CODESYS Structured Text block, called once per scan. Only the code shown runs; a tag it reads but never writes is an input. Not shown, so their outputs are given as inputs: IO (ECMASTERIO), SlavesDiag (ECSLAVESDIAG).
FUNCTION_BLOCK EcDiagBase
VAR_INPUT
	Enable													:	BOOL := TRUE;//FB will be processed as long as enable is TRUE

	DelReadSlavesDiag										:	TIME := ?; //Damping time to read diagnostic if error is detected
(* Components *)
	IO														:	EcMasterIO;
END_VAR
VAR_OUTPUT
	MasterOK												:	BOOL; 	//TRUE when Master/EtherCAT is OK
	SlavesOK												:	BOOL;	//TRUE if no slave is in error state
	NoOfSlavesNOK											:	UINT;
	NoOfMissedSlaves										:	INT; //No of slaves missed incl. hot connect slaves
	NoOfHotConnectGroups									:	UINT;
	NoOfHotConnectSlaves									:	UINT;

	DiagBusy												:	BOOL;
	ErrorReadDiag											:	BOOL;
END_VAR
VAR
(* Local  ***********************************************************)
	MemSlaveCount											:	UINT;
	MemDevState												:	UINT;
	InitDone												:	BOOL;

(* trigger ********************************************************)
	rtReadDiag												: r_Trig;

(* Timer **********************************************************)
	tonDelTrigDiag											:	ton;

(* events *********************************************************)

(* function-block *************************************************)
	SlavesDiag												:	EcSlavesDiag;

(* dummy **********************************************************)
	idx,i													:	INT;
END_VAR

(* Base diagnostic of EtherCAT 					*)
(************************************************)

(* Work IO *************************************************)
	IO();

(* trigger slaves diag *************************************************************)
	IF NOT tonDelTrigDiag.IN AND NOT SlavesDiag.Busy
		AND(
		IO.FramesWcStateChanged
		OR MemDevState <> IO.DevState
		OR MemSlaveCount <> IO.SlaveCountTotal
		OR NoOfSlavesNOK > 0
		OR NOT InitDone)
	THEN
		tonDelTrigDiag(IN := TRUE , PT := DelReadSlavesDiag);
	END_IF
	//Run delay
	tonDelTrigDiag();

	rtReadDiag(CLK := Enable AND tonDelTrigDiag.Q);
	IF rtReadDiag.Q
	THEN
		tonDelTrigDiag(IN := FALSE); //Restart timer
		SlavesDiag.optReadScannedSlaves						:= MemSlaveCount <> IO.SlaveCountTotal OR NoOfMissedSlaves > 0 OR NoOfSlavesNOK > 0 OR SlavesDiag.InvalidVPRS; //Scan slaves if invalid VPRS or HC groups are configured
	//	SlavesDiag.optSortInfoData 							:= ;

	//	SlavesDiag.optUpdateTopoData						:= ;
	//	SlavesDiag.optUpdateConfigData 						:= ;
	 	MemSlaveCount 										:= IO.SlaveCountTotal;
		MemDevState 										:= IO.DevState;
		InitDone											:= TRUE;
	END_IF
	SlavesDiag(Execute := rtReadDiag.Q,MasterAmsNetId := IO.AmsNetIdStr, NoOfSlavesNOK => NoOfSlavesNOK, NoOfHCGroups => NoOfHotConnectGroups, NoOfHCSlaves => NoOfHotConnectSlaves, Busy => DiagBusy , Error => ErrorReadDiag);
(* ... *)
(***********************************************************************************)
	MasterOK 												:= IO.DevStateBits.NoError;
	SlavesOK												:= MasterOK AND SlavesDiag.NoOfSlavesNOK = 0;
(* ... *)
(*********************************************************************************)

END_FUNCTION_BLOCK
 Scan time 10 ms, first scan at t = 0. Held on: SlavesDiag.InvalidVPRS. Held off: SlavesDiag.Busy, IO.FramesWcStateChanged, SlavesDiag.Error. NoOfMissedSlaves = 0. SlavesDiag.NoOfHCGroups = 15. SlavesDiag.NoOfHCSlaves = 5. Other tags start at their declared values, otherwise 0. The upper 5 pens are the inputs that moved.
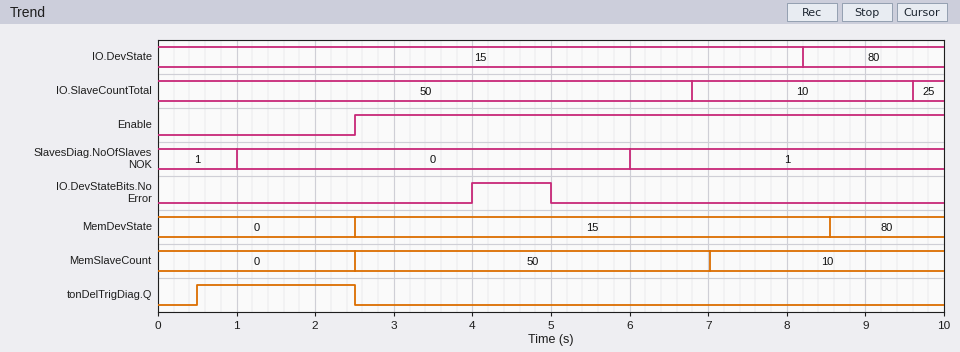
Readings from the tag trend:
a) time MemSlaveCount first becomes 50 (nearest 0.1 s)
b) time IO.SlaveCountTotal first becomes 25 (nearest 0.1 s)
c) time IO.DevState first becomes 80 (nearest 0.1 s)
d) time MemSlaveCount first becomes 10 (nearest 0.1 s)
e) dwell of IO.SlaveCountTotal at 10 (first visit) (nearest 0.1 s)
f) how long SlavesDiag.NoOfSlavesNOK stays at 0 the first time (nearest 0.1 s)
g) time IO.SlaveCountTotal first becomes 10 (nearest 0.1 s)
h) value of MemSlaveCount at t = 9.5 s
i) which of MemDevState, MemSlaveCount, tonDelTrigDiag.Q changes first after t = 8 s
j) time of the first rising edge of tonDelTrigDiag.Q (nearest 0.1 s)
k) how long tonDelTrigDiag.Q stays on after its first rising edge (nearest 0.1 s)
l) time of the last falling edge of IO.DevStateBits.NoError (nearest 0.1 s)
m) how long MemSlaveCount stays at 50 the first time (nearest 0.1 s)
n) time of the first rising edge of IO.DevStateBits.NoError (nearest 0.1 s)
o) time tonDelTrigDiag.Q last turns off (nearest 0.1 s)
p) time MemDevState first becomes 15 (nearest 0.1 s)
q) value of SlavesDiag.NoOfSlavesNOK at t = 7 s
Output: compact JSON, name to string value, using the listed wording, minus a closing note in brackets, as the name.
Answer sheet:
{"time MemSlaveCount first becomes 50": "2.5 s", "time IO.SlaveCountTotal first becomes 25": "9.6 s", "time IO.DevState first becomes 80": "8.2 s", "time MemSlaveCount first becomes 10": "7.0 s", "dwell of IO.SlaveCountTotal at 10 (first visit)": "2.8 s", "how long SlavesDiag.NoOfSlavesNOK stays at 0 the first time": "5.0 s", "time IO.SlaveCountTotal first becomes 10": "6.8 s", "value of MemSlaveCount at t = 9.5 s": "10", "which of MemDevState, MemSlaveCount, tonDelTrigDiag.Q changes first after t = 8 s": "MemDevState", "time of the first rising edge of tonDelTrigDiag.Q": "0.5 s", "how long tonDelTrigDiag.Q stays on after its first rising edge": "2.0 s", "time of the last falling edge of IO.DevStateBits.NoError": "5.0 s", "how long MemSlaveCount stays at 50 the first time": "4.5 s", "time of the first rising edge of IO.DevStateBits.NoError": "4.0 s", "time tonDelTrigDiag.Q last turns off": "2.5 s", "time MemDevState first becomes 15": "2.5 s", "value of SlavesDiag.NoOfSlavesNOK at t = 7 s": "1"}
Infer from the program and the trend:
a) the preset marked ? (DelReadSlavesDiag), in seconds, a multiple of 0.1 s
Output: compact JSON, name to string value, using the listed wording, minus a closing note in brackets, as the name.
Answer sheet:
{"the preset marked ? (DelReadSlavesDiag), in seconds, a multiple of 0.1 s": "0.5 s"}
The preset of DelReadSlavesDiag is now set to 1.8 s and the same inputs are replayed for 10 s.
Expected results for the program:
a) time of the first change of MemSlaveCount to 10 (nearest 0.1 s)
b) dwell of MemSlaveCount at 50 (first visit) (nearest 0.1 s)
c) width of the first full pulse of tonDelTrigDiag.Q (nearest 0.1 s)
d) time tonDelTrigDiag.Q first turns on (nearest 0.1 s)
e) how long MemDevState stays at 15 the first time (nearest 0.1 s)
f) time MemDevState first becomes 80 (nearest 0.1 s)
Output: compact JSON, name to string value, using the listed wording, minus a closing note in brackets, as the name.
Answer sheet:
{"time of the first change of MemSlaveCount to 10": "7.8 s", "dwell of MemSlaveCount at 50 (first visit)": "5.3 s", "width of the first full pulse of tonDelTrigDiag.Q": "0.7 s", "time tonDelTrigDiag.Q first turns on": "1.8 s", "how long MemDevState stays at 15 the first time": "7.1 s", "time MemDevState first becomes 80": "9.6 s"}
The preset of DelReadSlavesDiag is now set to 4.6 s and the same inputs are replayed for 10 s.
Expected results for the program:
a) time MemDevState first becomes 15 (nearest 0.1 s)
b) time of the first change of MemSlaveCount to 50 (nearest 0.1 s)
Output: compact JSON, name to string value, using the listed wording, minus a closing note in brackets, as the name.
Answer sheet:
{"time MemDevState first becomes 15": "4.6 s", "time of the first change of MemSlaveCount to 50": "4.6 s"}
